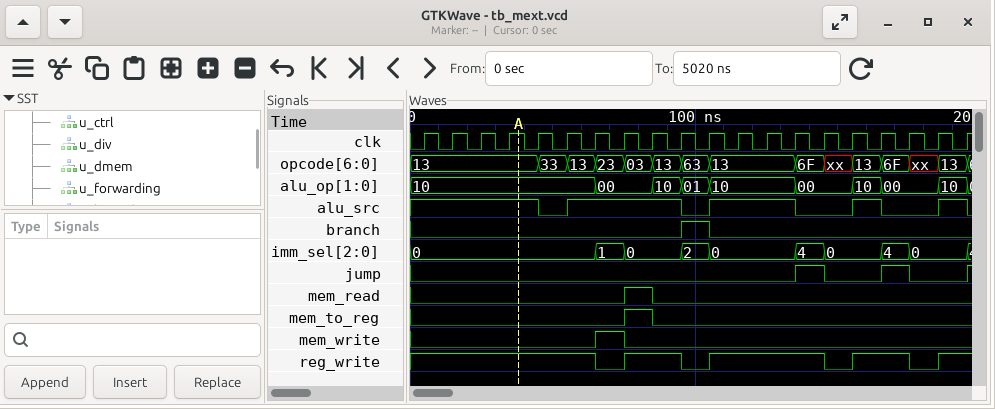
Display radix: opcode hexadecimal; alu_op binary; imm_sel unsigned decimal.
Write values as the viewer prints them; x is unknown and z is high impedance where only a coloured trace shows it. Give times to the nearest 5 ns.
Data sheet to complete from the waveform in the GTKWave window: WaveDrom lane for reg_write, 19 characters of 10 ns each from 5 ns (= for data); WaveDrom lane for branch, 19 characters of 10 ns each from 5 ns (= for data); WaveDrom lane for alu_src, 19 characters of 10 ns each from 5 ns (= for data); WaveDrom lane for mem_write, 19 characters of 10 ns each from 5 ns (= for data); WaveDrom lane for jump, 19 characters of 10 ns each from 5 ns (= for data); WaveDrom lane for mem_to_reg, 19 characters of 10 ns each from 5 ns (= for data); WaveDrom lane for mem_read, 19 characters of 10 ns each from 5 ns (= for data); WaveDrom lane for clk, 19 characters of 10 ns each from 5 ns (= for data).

{name: 'reg_write', wave: '1.....01.01...01.01'}
{name: 'branch', wave: '0........10........'}
{name: 'alu_src', wave: '1...01...01..0.10.1'}
{name: 'mem_write', wave: '0.....10...........'}
{name: 'jump', wave: '0............10.10.'}
{name: 'mem_to_reg', wave: '0......10..........'}
{name: 'mem_read', wave: '0......10..........'}
{name: 'clk', wave: 'p..................'}
